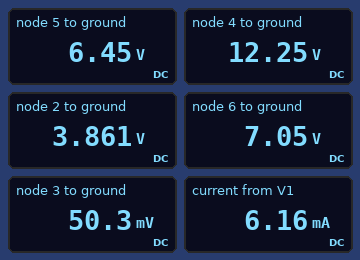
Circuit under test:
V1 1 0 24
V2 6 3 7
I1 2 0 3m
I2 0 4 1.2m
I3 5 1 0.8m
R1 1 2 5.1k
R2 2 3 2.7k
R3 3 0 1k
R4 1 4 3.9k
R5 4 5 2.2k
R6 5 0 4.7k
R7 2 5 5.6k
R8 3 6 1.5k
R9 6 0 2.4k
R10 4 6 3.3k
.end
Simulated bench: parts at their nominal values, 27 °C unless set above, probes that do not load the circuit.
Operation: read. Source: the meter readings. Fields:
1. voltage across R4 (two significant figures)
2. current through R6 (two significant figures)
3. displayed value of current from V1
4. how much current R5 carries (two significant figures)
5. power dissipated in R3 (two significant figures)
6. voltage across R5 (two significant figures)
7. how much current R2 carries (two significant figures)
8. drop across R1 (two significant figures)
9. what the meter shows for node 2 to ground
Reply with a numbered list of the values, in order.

1. 12 V
2. 1.4 mA
3. 6.16 mA
4. 2.6 mA
5. 2.5 µW
6. 5.8 V
7. 1.4 mA
8. 20 V
9. 3.861 V
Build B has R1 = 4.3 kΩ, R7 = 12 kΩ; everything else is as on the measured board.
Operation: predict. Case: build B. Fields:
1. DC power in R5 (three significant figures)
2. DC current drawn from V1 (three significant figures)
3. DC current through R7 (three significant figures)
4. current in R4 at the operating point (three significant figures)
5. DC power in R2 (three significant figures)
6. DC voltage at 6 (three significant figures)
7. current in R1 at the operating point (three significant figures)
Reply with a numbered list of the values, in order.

1. 13.8 mW
2. 6.60 mA
3. 194 µA
4. 2.92 mA
5. 7.51 mW
6. 7.26 V
7. 4.47 mA
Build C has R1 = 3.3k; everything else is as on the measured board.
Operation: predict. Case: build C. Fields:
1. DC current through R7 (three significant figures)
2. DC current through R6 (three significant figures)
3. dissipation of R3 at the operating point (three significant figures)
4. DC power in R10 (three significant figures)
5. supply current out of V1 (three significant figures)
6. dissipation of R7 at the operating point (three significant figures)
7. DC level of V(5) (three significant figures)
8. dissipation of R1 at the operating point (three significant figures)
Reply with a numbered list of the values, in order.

1. 99.5 µA
2. 1.58 mA
3. 451 µW
4. 8.19 mW
5. 7.25 mA
6. 55.4 µW
7. 7.42 V
8. 89.0 mW
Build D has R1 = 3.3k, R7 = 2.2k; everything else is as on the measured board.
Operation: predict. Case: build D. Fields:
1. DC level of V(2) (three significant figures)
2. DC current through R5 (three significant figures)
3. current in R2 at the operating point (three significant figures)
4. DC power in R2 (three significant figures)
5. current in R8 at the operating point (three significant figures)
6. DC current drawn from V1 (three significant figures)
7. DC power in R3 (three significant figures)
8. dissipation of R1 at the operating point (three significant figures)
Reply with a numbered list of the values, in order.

1. 6.95 V
2. 2.51 mA
3. 2.32 mA
4. 14.6 mW
5. 4.67 mA
6. 7.23 mA
7. 463 µW
8. 88.1 mW
